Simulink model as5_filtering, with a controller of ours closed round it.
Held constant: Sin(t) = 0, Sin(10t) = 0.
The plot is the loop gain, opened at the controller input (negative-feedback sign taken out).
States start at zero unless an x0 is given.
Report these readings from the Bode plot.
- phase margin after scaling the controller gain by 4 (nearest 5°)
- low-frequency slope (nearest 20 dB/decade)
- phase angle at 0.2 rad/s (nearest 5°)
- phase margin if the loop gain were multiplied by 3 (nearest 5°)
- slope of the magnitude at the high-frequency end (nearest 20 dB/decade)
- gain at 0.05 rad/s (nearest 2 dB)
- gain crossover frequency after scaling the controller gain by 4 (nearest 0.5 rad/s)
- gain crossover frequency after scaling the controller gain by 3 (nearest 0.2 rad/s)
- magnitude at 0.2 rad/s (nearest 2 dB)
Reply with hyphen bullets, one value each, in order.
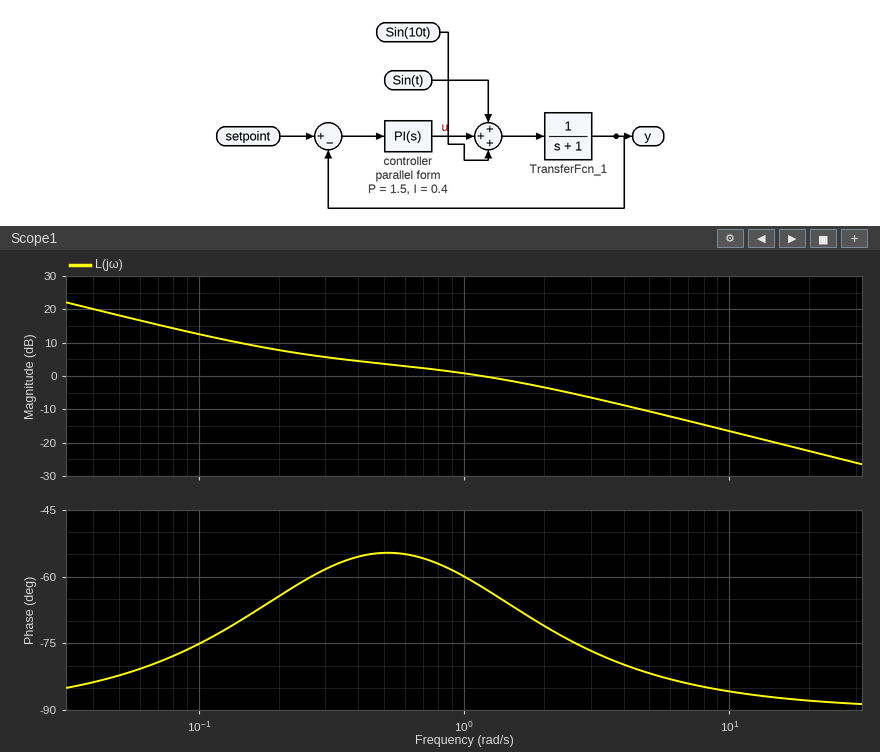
- 95°
- -20 dB/decade
- -65°
- 100°
- -20 dB/decade
- 18 dB
- 6.0 rad/s
- 4.4 rad/s
- 8 dB
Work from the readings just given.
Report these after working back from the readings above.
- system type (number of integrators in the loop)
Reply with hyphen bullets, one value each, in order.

- 1
